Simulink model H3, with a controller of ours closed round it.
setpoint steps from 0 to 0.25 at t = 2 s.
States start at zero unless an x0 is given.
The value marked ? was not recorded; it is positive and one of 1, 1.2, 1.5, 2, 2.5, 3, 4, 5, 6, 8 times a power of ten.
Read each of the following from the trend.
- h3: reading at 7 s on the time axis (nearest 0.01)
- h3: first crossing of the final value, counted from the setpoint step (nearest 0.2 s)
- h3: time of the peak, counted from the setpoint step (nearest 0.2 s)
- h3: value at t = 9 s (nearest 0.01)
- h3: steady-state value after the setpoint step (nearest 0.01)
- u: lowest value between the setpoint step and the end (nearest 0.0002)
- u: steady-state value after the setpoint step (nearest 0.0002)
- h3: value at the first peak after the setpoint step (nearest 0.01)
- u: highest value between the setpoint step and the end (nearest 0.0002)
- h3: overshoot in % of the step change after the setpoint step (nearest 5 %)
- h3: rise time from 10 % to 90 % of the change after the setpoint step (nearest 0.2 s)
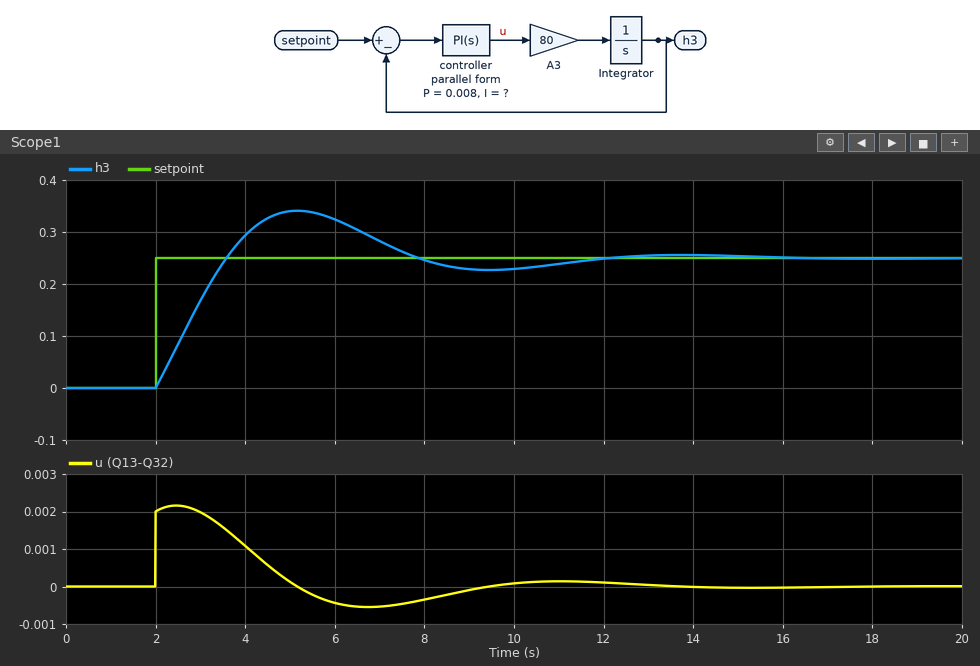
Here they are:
0.28
1.6 s
3.2 s
0.23
0.25
-0.0006
0.0000
0.34
0.0022
35 %
1.2 s
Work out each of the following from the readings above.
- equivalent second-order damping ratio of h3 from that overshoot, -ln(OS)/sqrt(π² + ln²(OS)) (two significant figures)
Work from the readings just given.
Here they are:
0.32
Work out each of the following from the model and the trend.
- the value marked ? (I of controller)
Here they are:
0.008
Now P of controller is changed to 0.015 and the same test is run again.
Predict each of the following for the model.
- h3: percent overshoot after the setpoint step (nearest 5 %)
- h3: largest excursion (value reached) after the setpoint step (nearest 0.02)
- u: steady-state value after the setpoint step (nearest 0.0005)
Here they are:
20 %
0.30
0.0000
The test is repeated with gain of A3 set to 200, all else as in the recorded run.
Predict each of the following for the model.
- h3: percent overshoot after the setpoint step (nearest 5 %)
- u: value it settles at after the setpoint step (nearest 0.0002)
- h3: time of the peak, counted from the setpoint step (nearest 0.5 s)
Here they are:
25 %
0.0000
2.0 s
